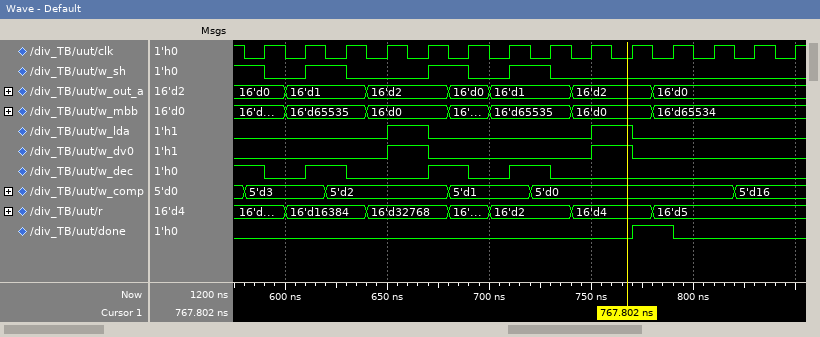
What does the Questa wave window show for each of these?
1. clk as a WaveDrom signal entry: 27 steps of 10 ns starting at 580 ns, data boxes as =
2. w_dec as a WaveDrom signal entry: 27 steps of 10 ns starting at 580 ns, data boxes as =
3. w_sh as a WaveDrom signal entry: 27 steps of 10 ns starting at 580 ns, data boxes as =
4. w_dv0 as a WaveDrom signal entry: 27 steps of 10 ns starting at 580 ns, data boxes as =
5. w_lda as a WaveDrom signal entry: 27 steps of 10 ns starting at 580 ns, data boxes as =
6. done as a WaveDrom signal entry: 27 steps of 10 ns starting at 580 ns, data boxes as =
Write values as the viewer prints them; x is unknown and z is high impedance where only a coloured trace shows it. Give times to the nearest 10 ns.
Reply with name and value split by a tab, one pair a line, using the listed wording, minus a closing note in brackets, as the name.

clk as a WaveDrom signal entry: 27 steps of 10 ns starting at 580 ns, data boxes as =	{name: 'clk', wave: '010101010101010101010101010'}
w_dec as a WaveDrom signal entry: 27 steps of 10 ns starting at 580 ns, data boxes as =	{name: 'w_dec', wave: '10.1.0...1.0.1.0...........'}
w_sh as a WaveDrom signal entry: 27 steps of 10 ns starting at 580 ns, data boxes as =	{name: 'w_sh', wave: '10.1.0...1.0.1.0...........'}
w_dv0 as a WaveDrom signal entry: 27 steps of 10 ns starting at 580 ns, data boxes as =	{name: 'w_dv0', wave: '0......1.0.......1.0.......'}
w_lda as a WaveDrom signal entry: 27 steps of 10 ns starting at 580 ns, data boxes as =	{name: 'w_lda', wave: '0......1.0.......1.0.......'}
done as a WaveDrom signal entry: 27 steps of 10 ns starting at 580 ns, data boxes as =	{name: 'done', wave: '0..................1.0.....'}
